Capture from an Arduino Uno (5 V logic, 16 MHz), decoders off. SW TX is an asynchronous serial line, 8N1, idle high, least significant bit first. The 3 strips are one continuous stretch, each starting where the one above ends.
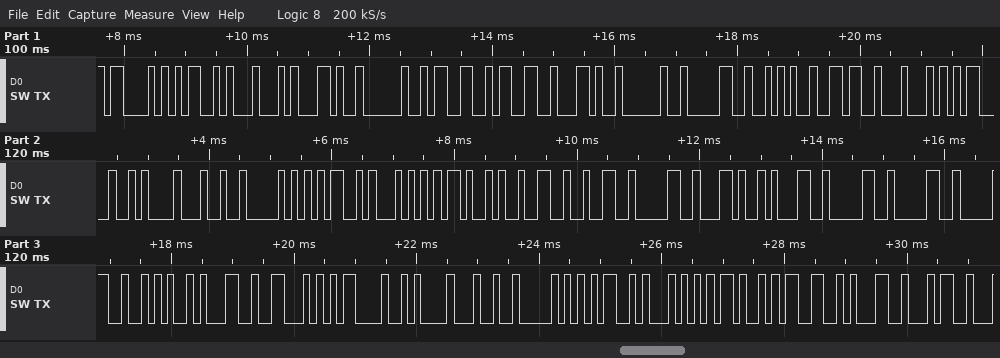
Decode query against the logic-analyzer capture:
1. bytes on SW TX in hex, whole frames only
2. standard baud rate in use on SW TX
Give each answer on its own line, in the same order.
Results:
0x43 0x4D 0x44 0x2C 0x20 0x33 0x33 0x2C 0x20 0x30 0x2A 0x36 0x44 0x0D 0x0A 0x24 0x50 0x4D 0x54 0x4B 0x32 0x32 0x30 0x2C 0x31 0x30 0x30 0x30 0x2A 0x31 0x46 0x0D 0x0A 0x24 0x50 0x4D 0x54 0x4B 0x33 0x31 0x34
9600 baud
